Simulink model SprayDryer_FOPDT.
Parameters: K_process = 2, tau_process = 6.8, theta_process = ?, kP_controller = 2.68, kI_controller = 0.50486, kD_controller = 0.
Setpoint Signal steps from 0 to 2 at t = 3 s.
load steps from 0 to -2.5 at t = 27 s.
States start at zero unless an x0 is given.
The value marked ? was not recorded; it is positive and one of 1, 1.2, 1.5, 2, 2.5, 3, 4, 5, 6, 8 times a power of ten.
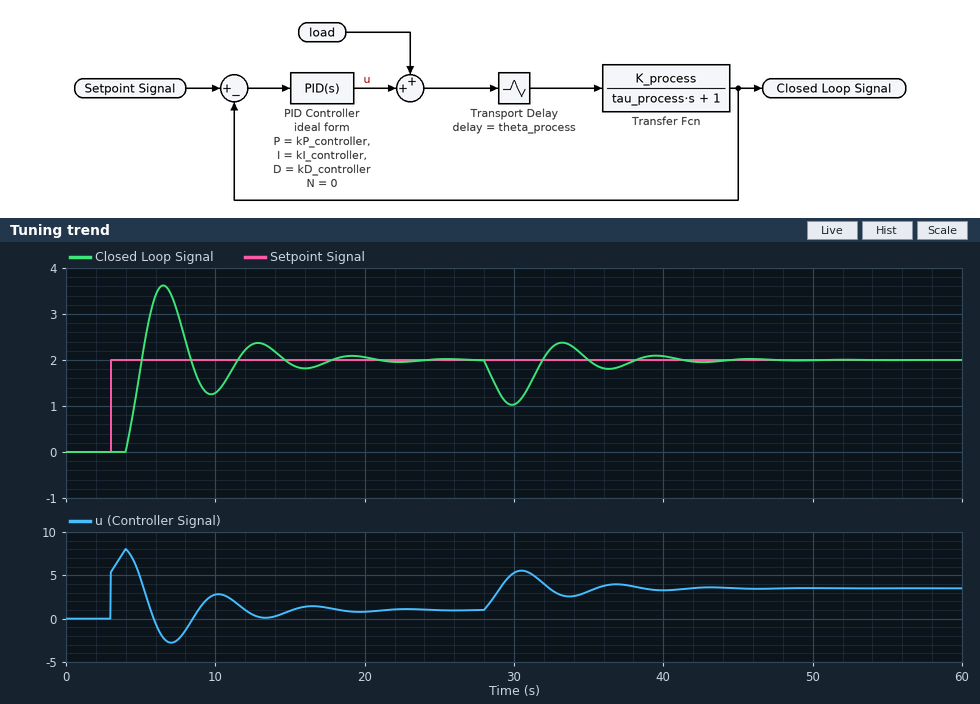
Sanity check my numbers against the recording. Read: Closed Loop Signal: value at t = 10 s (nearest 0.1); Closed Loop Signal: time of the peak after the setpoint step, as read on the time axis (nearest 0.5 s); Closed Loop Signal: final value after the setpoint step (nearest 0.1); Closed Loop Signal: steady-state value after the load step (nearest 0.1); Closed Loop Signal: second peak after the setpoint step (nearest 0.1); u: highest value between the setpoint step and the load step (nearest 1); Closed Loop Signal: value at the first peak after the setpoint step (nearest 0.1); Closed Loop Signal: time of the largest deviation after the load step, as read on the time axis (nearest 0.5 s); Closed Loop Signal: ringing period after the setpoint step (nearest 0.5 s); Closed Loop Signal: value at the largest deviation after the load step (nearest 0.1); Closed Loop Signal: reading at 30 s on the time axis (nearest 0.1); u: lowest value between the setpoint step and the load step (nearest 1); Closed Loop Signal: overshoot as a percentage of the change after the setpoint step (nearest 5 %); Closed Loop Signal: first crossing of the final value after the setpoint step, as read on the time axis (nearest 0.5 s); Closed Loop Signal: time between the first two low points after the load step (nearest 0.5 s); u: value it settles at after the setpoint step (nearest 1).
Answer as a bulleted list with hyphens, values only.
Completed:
- 1.3
- 6.5 s
- 2.0
- 2.0
- 2.4
- 8
- 3.6
- 30.0 s
- 6.5 s
- 1.0
- 1.0
- -3
- 80 %
- 5.0 s
- 6.5 s
- 1
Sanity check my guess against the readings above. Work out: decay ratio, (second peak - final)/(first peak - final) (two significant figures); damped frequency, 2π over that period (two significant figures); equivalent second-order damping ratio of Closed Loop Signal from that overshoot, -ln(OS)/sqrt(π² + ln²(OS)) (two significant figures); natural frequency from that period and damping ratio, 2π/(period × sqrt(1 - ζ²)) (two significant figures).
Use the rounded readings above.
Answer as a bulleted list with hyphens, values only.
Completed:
- 0.25
- 0.97 rad/s
- 0.071
- 0.97 rad/s
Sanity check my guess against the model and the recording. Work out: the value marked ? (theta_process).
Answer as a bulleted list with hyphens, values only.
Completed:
- 1
